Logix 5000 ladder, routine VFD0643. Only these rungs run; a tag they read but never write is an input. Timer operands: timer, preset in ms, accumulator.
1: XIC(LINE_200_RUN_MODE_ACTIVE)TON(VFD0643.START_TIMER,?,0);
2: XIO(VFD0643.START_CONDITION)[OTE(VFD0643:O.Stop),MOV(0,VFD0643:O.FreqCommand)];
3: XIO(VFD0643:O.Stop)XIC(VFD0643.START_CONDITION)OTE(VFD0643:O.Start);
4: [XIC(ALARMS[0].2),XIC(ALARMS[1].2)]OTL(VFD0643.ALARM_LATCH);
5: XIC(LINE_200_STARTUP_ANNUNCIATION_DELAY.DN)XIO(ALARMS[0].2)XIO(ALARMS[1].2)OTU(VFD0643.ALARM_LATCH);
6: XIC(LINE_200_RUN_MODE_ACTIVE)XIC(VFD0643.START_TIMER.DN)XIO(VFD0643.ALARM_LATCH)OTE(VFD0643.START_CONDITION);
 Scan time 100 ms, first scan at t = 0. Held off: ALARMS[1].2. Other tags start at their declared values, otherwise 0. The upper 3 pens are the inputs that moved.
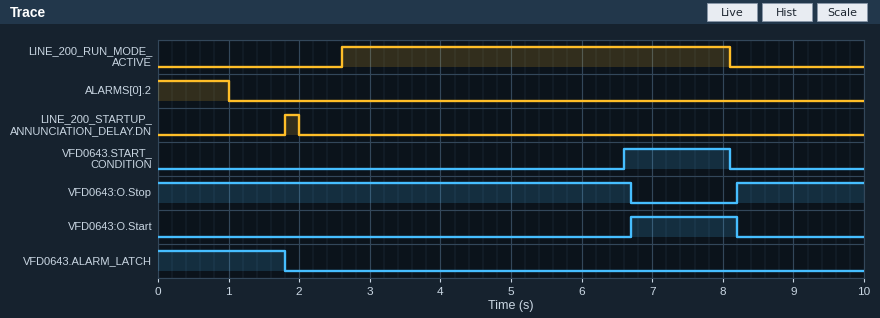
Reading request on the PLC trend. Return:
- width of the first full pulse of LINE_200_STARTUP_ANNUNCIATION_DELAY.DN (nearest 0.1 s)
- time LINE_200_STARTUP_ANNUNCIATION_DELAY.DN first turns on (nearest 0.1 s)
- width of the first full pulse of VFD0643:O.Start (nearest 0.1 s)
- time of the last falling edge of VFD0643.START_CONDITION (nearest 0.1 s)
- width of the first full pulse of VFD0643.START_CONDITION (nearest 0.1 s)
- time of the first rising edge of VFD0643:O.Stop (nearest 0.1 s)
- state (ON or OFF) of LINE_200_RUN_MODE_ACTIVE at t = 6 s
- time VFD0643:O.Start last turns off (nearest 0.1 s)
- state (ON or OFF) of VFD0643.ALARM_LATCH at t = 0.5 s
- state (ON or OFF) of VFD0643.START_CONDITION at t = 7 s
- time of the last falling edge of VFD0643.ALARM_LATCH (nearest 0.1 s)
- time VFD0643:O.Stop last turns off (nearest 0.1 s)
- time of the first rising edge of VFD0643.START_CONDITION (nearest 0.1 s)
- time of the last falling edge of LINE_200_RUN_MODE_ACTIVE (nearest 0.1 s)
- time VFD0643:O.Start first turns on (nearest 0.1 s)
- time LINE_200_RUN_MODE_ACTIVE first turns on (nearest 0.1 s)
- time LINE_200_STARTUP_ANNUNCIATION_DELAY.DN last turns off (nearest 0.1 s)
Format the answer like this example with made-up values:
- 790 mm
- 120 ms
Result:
- 0.2 s
- 1.8 s
- 1.5 s
- 8.1 s
- 1.5 s
- 8.2 s
- ON
- 8.2 s
- ON
- ON
- 1.8 s
- 6.7 s
- 6.6 s
- 8.1 s
- 6.7 s
- 2.6 s
- 2.0 s
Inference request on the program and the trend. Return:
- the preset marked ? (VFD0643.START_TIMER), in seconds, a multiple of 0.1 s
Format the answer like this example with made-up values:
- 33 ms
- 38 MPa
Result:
- 4.0 s
